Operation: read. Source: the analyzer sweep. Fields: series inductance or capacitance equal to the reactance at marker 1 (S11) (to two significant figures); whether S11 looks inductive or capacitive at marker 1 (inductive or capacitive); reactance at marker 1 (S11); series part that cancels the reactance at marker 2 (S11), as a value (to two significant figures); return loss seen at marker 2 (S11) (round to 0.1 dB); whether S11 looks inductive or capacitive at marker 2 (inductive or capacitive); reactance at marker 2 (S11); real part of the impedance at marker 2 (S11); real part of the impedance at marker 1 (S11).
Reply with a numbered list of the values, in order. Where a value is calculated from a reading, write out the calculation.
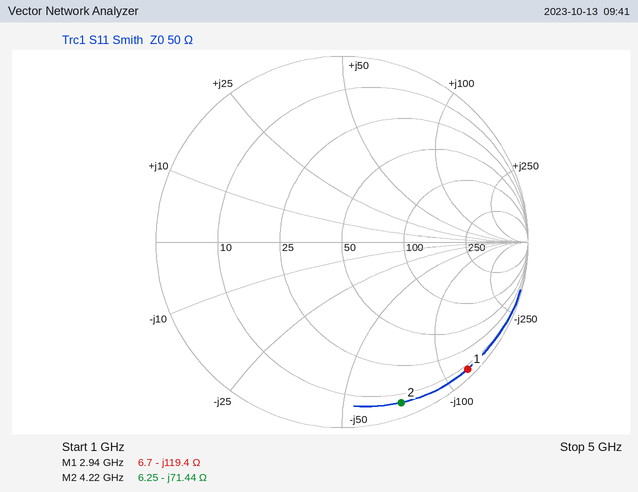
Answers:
1. C = 1/(2π × 2.94 GHz × 119.4 Ω) ≈ 453 fF, so 450 fF to two significant figures
2. capacitive
3. -119.4 Ω
4. L = 71.44 Ω/(2π × 4.22 GHz) ≈ 2.7 nH
5. 0.7 dB
6. capacitive
7. -71.44 Ω
8. 6.25 Ω
9. 6.7 Ω
